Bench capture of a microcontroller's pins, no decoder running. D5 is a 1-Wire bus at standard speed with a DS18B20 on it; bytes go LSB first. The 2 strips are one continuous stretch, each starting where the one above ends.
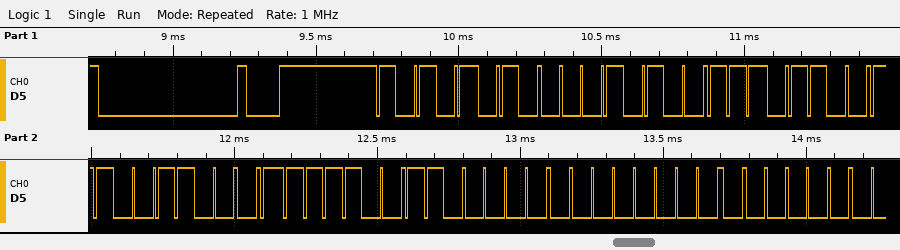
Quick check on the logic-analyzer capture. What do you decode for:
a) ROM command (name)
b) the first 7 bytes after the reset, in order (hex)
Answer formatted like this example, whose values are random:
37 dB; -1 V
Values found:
Match ROM; 55 28 37 33 3E 03 00
